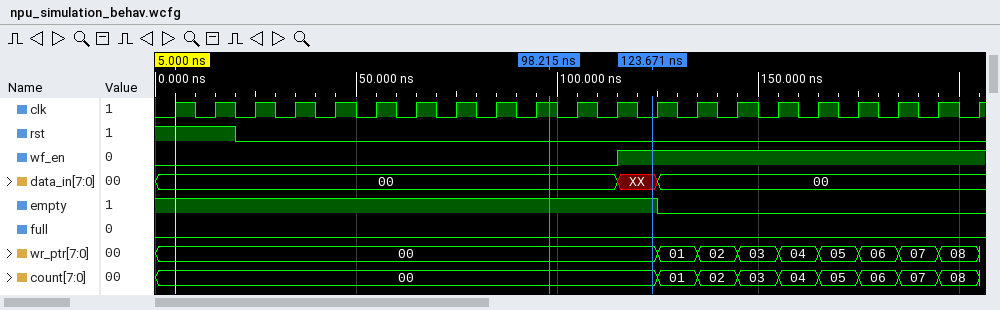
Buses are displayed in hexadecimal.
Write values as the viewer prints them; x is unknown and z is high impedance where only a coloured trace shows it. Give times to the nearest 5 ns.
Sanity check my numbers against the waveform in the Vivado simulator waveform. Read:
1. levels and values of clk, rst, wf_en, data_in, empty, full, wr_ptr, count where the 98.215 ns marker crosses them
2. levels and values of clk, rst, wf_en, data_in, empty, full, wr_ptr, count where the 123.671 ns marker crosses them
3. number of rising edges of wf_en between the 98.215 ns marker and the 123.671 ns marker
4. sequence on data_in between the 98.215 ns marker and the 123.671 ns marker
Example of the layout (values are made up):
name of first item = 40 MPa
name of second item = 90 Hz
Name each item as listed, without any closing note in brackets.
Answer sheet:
levels and values of clk, rst, wf_en, data_in, empty, full, wr_ptr, count where the 98.215 ns marker crosses them = clk=1, rst=0, wf_en=0, data_in=00, empty=1, full=0, wr_ptr=00, count=00
levels and values of clk, rst, wf_en, data_in, empty, full, wr_ptr, count where the 123.671 ns marker crosses them = clk=0, rst=0, wf_en=1, data_in=XX, empty=1, full=0, wr_ptr=00, count=00
number of rising edges of wf_en between the 98.215 ns marker and the 123.671 ns marker = 1
sequence on data_in between the 98.215 ns marker and the 123.671 ns marker = 00, XX
